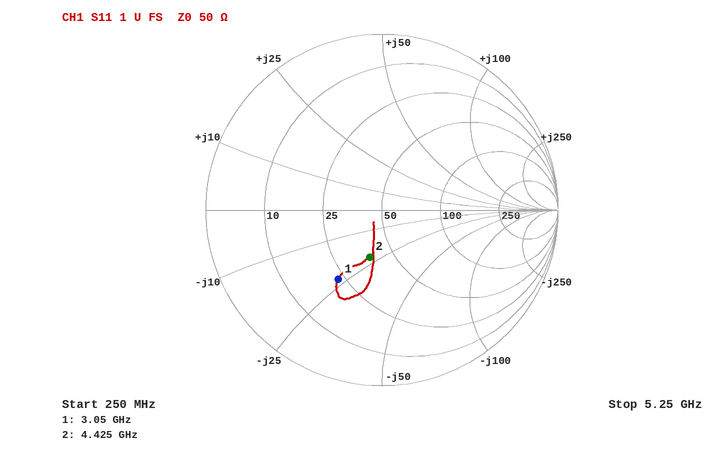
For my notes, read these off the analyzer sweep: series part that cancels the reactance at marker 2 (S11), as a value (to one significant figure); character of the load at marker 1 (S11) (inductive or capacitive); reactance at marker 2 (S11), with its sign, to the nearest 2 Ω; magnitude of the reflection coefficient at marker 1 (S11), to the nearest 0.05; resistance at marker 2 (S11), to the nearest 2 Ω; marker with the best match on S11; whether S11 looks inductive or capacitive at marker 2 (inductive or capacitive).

800 pH
capacitive
-22 Ω
0.45
38 Ω
marker 2
capacitive
